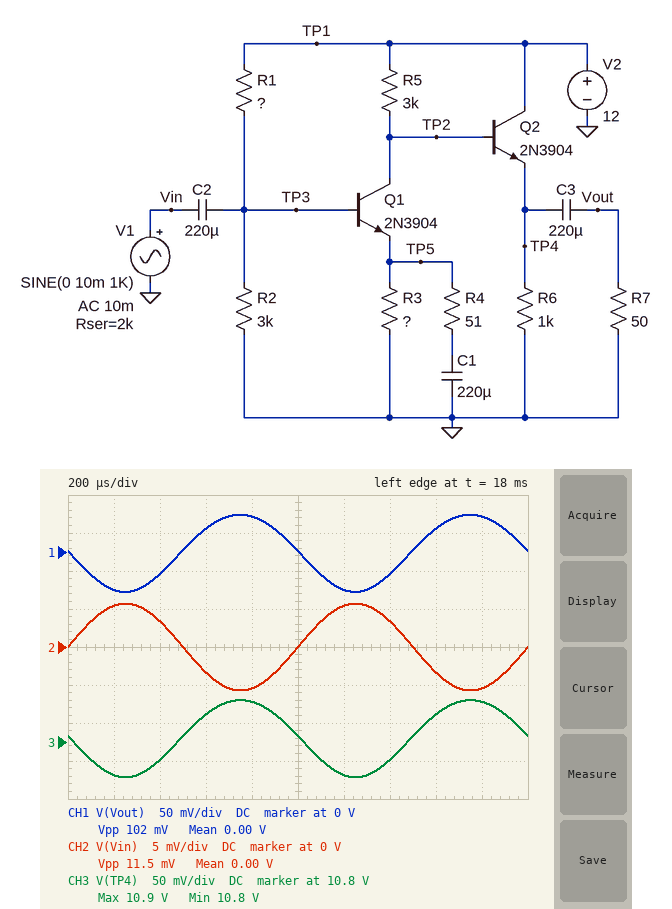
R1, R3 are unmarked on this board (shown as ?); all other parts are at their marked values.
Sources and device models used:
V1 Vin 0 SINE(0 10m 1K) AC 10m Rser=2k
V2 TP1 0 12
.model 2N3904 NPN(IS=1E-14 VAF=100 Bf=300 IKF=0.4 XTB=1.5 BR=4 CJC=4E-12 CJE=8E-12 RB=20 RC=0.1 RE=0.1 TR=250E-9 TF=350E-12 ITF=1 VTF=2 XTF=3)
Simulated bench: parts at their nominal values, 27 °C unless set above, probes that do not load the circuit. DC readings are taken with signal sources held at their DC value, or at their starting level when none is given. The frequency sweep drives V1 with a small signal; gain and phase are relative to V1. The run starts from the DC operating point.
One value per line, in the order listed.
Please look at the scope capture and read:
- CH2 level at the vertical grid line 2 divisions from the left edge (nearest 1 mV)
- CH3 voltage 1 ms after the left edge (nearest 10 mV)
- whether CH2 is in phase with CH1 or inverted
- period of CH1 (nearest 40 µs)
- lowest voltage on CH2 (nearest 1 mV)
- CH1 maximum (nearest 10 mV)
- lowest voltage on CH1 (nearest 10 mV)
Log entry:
3 mV
10.81 V
inverted
1.00 ms
-6 mV
50 mV
-50 mV
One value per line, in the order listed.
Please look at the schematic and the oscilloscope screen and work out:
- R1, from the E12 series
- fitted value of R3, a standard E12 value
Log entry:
33 kΩ
3.3 kΩ
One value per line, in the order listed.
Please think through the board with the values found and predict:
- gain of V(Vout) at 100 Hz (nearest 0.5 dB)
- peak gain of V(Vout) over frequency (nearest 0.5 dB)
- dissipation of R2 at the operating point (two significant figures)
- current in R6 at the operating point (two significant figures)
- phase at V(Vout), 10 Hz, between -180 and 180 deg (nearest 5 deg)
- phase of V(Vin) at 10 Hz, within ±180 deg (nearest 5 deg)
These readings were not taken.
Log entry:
14.0 dB
14.0 dB
330 µW
11 mA
-115 deg
0 deg
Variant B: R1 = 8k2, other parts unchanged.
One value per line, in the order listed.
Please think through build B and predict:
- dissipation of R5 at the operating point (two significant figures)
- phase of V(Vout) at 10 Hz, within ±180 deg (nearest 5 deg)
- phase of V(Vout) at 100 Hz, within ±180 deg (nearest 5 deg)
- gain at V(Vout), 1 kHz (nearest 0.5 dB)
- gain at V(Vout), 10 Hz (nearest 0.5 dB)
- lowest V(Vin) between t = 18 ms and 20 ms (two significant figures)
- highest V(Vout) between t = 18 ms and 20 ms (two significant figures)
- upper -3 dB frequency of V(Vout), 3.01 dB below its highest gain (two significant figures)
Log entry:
1.9 mW
-90 deg
-170 deg
23.0 dB
17.0 dB
-5.0 mV
140 mV
1.7 MHz
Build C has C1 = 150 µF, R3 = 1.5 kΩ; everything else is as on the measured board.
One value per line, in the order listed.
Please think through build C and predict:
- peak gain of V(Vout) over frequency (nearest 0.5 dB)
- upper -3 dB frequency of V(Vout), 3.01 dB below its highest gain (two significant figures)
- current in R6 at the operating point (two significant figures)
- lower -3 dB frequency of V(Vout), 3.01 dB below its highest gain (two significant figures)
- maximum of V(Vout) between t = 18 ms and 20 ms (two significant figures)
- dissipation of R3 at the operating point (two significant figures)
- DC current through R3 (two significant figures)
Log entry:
19.0 dB
2.3 MHz
10 mA
15 Hz
85 mV
97 µW
250 µA
